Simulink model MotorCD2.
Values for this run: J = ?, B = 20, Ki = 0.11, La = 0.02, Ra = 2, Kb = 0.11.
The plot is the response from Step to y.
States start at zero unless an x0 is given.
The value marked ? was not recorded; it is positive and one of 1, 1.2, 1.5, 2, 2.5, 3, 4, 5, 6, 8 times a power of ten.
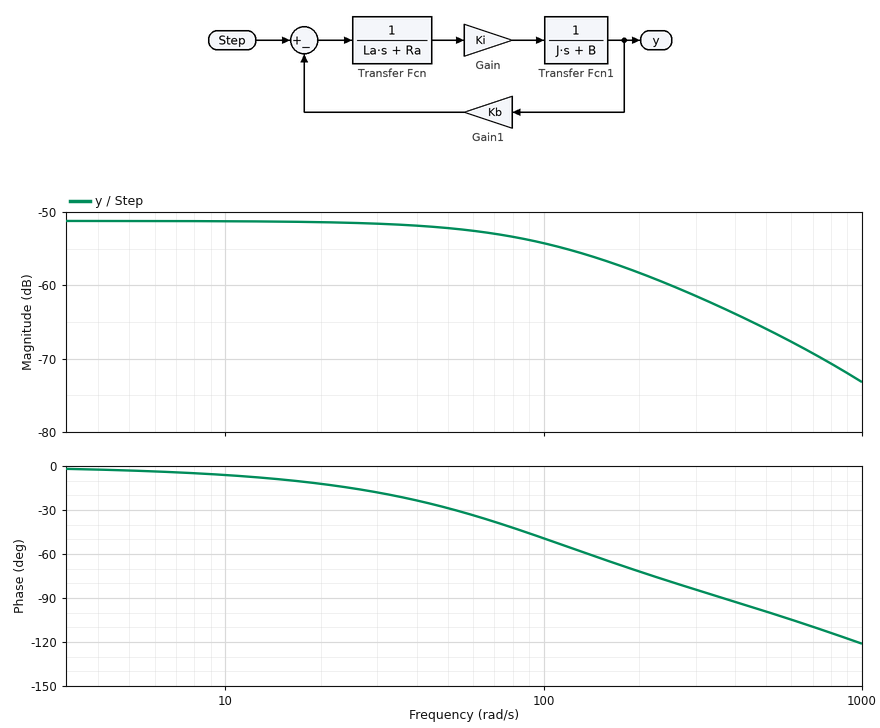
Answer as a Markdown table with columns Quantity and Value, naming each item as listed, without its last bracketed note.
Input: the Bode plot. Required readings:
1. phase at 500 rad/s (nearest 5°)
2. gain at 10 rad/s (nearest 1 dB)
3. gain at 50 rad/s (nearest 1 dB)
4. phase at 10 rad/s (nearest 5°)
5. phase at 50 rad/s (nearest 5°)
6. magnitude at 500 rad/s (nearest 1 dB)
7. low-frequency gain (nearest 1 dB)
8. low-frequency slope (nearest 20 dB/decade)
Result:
| Quantity | Value |
|---|---|
| phase at 500 rad/s | -100° |
| gain at 10 rad/s | -51 dB |
| gain at 50 rad/s | -52 dB |
| phase at 10 rad/s | -5° |
| phase at 50 rad/s | -30° |
| magnitude at 500 rad/s | -66 dB |
| low-frequency gain | -51 dB |
| low-frequency slope | 0 dB/decade |
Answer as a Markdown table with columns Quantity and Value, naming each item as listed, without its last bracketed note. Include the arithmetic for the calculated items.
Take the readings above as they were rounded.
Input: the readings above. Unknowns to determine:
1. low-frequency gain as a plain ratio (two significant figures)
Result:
| Quantity | Value |
|---|---|
| low-frequency gain as a plain ratio | 10^(-51 / 20) = 0.0028 |
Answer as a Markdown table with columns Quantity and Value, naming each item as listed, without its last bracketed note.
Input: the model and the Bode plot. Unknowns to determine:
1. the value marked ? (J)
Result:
| Quantity | Value |
|---|---|
| the value marked ? | 0.015 |
